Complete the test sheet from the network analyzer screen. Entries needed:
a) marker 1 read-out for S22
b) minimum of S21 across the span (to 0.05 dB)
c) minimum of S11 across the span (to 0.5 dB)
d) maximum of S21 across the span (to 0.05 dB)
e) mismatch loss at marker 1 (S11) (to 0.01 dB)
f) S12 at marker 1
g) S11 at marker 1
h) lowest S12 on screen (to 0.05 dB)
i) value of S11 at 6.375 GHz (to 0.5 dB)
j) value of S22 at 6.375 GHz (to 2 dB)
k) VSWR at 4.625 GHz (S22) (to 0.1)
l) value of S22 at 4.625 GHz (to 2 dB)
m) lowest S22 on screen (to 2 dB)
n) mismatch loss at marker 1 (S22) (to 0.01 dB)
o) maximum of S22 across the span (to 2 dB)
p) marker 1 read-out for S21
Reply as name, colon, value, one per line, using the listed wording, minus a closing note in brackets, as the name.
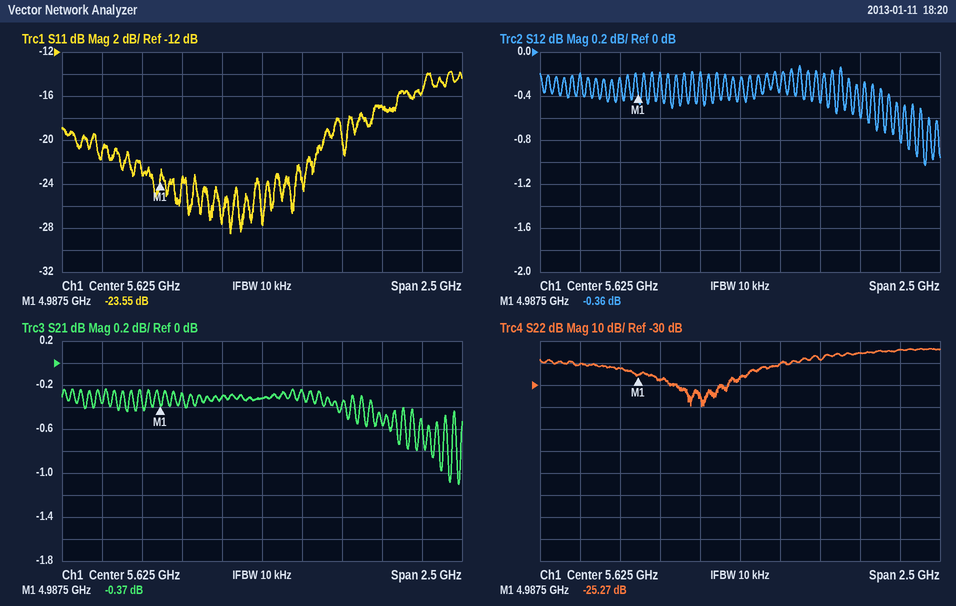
marker 1 read-out for S22: -25.27 dB
minimum of S21 across the span: -1.10 dB
minimum of S11 across the span: -28.5 dB
maximum of S21 across the span: -0.25 dB
mismatch loss at marker 1 (S11): 0.02 dB
S12 at marker 1: -0.36 dB
S11 at marker 1: -23.55 dB
lowest S12 on screen: -1.05 dB
value of S11 at 6.375 GHz: -17.0 dB
value of S22 at 6.375 GHz: -16 dB
VSWR at 4.625 GHz (S22): 1.2
value of S22 at 4.625 GHz: -20 dB
lowest S22 on screen: -40 dB
mismatch loss at marker 1 (S22): 0.01 dB
maximum of S22 across the span: -14 dB
marker 1 read-out for S21: -0.37 dB
